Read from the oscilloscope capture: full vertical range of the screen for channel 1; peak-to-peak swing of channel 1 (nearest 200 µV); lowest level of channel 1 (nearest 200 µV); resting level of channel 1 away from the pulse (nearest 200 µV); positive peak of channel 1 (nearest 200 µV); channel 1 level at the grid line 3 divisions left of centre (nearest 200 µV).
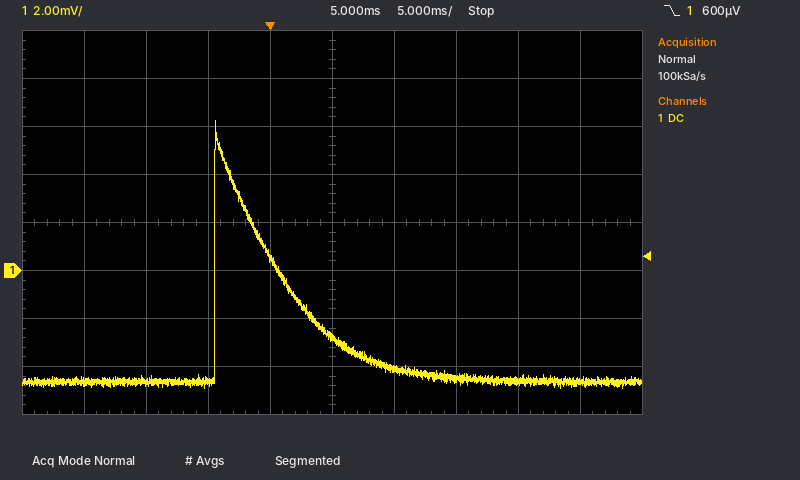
16 mV
11.2 mV
-5.0 mV
-4.6 mV
6.2 mV
-4.6 mV
